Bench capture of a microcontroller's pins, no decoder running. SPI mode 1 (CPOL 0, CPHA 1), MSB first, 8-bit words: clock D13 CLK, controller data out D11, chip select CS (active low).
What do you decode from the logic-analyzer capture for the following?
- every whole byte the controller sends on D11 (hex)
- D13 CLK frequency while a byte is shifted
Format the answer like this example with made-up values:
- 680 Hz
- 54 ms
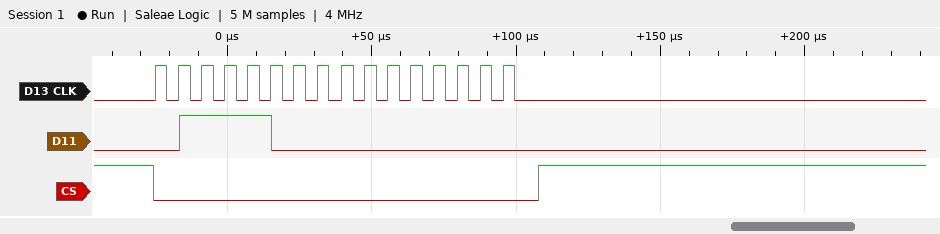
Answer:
- 78 00
- 125 kHz
